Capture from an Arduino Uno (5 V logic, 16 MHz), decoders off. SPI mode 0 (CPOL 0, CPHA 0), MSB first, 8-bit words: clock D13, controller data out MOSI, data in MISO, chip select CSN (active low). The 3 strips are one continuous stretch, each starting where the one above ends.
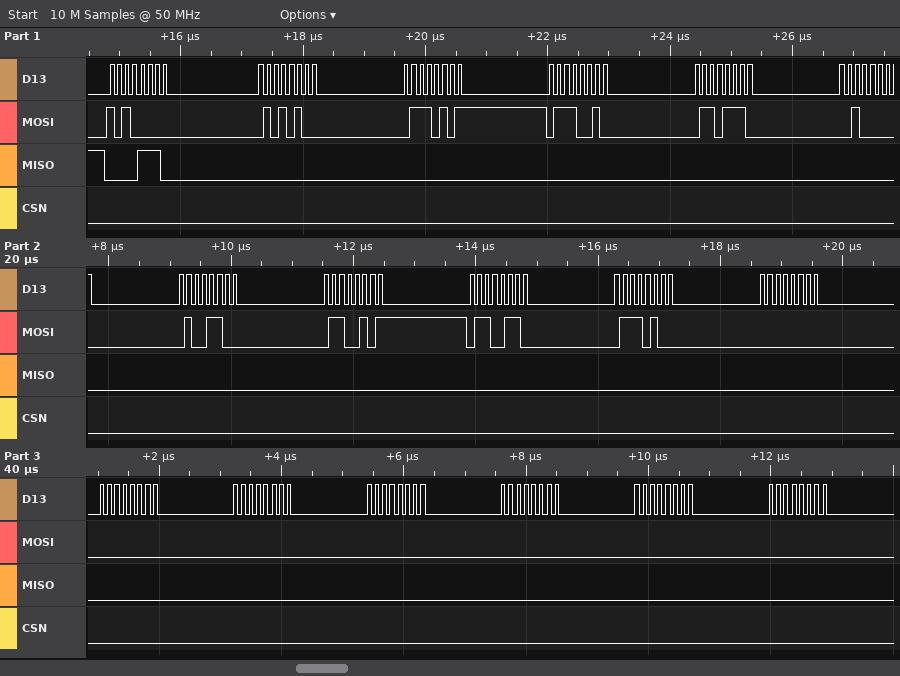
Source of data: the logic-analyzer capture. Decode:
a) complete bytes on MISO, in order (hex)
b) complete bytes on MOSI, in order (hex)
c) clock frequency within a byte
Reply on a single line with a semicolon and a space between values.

0x0E 0x00 0x00 0x00 0x00 0x00 0x00 0x00 0x00 0x00 0x00 0x00 0x00 0x00 0x00 0x00 0x00; 0xA0 0x54 0x75 0x72 0x6E 0x20 0x4C 0x65 0x66 0x74 0x00 0x00 0x00 0x00 0x00 0x00 0x00; 8 MHz
